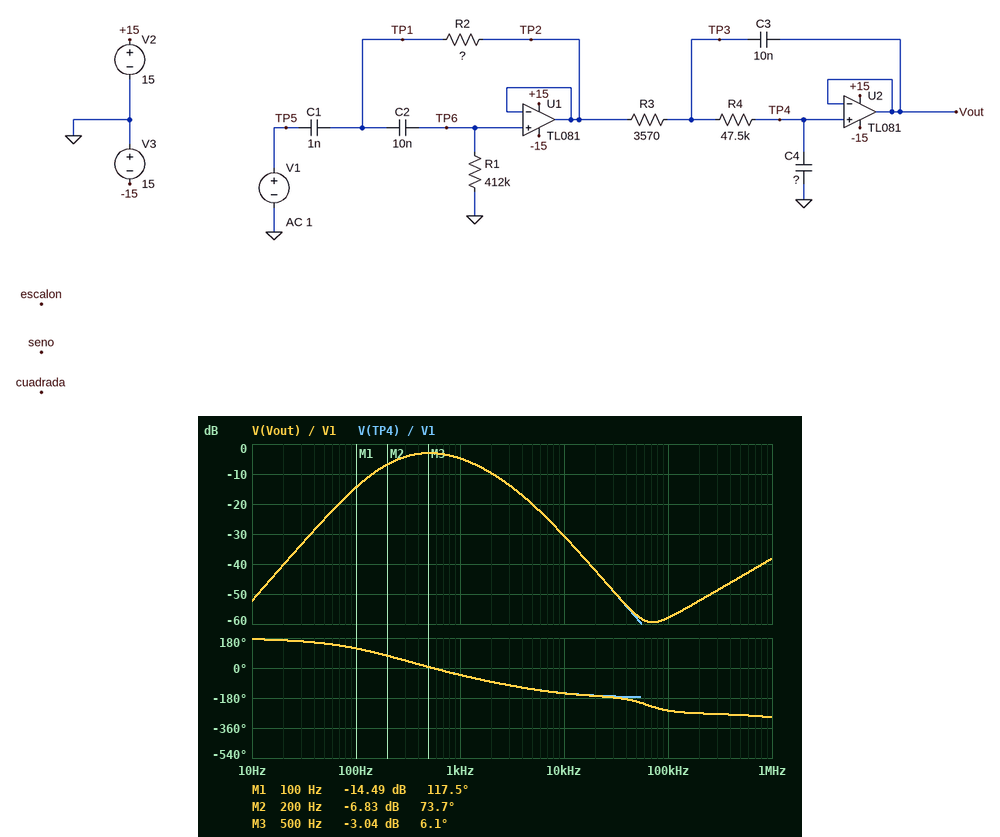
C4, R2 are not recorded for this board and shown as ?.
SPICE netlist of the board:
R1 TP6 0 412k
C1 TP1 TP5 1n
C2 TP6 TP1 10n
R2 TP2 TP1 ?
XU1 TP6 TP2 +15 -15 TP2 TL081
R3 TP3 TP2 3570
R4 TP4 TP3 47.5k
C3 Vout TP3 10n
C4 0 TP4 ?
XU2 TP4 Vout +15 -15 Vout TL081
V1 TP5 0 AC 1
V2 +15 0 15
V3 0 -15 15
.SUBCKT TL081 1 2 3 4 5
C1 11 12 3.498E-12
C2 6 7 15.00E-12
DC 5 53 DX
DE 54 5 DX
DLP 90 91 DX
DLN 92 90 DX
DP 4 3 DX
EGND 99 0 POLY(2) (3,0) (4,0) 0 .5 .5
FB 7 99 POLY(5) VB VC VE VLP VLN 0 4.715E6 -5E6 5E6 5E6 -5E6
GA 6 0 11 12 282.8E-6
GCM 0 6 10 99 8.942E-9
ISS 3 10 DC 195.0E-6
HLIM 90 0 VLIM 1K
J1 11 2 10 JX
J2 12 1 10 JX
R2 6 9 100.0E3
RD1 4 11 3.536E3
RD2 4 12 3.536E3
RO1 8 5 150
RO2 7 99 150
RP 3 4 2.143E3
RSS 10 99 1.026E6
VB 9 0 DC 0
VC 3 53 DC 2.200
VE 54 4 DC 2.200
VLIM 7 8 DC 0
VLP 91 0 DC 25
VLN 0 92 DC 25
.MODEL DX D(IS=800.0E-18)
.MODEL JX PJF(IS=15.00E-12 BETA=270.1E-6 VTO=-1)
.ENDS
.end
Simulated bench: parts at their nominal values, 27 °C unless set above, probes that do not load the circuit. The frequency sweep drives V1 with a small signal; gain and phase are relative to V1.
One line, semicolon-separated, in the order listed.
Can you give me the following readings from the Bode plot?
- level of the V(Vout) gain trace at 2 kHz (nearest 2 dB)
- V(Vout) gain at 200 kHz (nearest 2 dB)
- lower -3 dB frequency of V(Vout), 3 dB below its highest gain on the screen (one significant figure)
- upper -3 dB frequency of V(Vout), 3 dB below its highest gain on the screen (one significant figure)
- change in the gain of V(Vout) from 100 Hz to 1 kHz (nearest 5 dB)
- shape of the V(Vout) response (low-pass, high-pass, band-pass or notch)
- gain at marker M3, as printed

-10 dB; -52 dB; 200 Hz; 1 kHz; 10 dB; band-pass; -3.04 dB
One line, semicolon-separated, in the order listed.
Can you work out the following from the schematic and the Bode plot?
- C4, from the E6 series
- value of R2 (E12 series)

4.7 nF; 150 kΩ
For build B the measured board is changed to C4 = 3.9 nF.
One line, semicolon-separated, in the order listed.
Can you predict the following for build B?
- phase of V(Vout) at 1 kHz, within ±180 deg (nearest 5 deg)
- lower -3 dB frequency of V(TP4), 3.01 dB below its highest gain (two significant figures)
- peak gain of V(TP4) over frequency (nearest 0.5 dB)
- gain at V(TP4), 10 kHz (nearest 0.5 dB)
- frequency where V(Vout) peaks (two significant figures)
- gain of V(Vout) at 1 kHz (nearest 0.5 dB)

-35 deg; 230 Hz; -2.5 dB; -29.0 dB; 560 Hz; -3.5 dB
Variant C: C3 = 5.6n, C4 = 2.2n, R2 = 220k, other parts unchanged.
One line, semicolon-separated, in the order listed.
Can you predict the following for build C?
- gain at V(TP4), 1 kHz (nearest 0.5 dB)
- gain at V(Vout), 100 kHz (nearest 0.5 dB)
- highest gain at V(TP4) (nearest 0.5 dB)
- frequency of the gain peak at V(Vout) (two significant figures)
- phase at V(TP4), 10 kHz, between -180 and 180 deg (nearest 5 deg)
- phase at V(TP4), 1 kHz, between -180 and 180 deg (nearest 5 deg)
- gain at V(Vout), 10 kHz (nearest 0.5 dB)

-2.0 dB; -55.5 dB; -1.5 dB; 780 Hz; -135 deg; -15 deg; -20.0 dB
